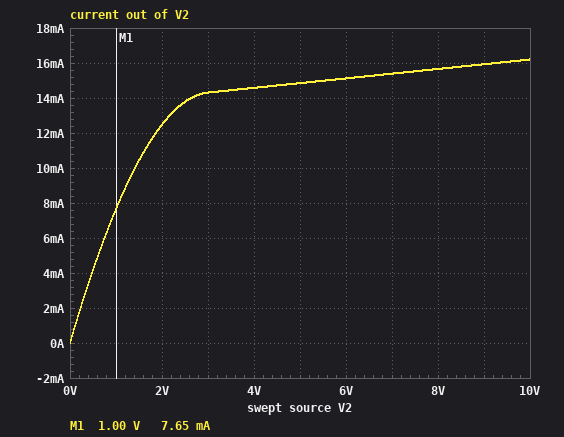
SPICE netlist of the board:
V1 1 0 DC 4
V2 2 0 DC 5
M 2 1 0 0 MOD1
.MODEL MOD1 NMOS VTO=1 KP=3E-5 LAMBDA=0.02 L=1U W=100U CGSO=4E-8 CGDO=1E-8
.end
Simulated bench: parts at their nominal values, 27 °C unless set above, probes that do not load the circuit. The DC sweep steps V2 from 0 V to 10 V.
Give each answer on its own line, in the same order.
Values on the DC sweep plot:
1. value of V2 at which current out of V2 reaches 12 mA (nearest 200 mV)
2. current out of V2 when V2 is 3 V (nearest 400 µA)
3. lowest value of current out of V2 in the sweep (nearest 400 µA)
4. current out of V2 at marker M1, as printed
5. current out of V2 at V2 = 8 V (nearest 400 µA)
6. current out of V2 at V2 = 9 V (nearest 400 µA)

1.8 V
14.4 mA
0 A
7.65 mA
15.6 mA
16.0 mA
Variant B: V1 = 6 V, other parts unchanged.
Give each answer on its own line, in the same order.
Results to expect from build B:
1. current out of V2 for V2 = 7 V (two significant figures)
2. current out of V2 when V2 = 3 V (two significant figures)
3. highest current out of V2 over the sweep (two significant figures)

43 mA
33 mA
45 mA
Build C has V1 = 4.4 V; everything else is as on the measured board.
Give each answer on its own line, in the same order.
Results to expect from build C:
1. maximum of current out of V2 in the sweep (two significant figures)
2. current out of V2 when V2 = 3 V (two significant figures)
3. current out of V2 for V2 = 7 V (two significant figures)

21 mA
18 mA
20 mA
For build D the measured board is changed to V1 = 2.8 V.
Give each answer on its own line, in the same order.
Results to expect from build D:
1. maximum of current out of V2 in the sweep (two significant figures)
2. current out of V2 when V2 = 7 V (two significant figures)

5.8 mA
5.5 mA
